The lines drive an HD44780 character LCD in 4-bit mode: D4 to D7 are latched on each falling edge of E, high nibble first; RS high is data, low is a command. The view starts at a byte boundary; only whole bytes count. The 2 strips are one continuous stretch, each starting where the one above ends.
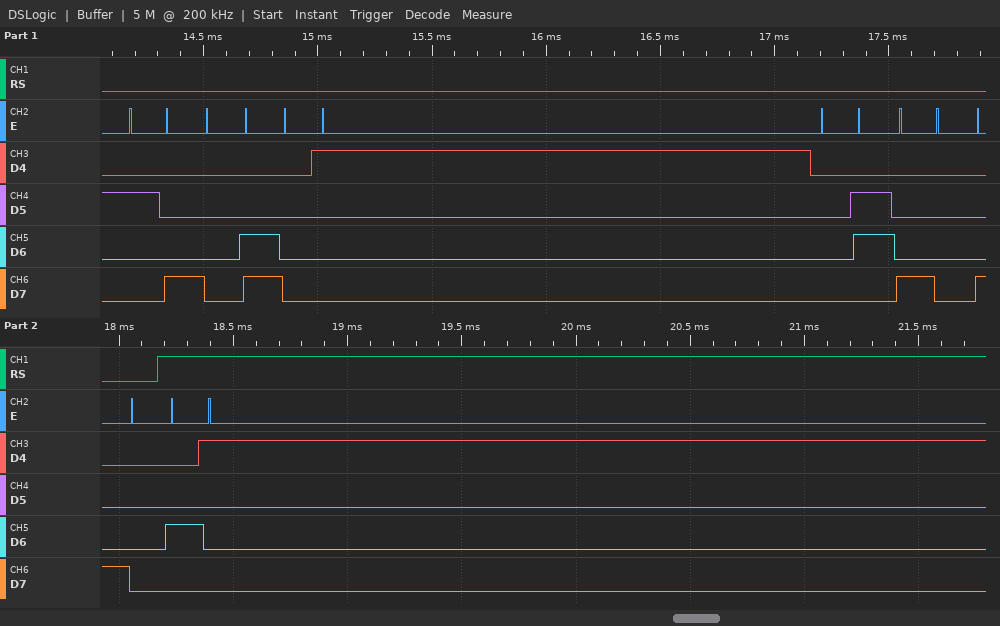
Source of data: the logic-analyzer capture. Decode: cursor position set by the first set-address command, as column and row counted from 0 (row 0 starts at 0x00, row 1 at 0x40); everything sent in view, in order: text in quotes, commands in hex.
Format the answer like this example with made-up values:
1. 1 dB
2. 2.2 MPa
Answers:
1. column 0, row 0
2. 0x28 0x0C 0x01 0x06 0x80 0x80 "A"
